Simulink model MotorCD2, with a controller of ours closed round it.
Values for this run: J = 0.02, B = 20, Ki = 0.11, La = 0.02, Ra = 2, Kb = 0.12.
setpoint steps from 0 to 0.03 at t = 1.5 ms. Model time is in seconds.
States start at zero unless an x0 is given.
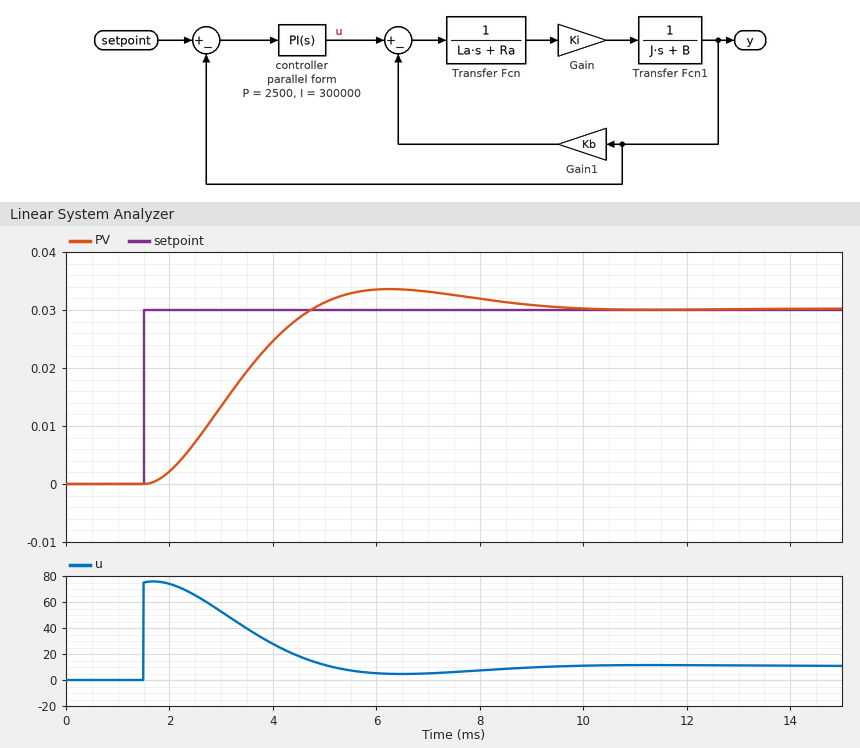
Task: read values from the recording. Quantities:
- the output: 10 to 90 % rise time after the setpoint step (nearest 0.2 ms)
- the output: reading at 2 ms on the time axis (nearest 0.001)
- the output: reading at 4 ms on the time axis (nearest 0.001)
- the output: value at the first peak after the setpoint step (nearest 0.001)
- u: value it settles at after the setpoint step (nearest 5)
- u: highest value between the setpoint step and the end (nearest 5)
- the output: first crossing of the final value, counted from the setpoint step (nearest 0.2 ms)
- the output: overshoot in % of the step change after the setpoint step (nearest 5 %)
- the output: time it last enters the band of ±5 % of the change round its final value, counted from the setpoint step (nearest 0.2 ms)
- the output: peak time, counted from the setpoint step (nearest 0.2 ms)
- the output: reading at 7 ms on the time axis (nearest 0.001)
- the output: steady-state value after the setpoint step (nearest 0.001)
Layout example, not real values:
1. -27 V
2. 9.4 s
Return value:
1. 2.2 ms
2. 0.002
3. 0.025
4. 0.034
5. 10
6. 75
7. 3.2 ms
8. 10 %
9. 6.8 ms
10. 4.8 ms
11. 0.033
12. 0.030
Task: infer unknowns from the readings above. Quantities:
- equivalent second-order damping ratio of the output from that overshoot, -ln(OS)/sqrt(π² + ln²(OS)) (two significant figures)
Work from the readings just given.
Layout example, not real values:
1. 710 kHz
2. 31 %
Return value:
1. 0.59
